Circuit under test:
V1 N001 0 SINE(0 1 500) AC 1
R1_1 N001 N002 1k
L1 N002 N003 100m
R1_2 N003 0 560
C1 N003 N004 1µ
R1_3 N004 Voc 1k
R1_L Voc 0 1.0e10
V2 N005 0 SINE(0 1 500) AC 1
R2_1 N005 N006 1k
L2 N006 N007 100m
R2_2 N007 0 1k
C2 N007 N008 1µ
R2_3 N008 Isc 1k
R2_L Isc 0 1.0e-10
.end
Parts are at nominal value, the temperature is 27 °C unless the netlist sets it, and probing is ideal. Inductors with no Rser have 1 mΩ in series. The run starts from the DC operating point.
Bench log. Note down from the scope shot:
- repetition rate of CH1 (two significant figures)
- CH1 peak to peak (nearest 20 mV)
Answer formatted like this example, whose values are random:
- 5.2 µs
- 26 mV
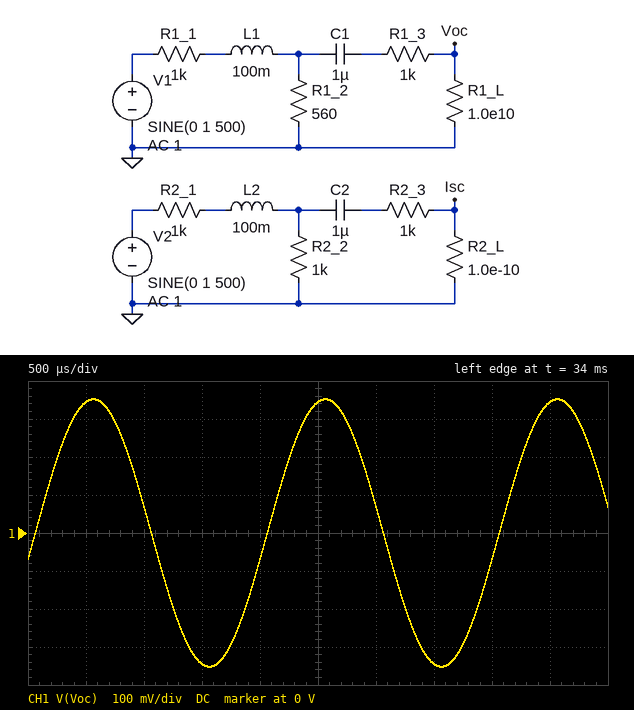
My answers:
- 500 Hz
- 700 mV
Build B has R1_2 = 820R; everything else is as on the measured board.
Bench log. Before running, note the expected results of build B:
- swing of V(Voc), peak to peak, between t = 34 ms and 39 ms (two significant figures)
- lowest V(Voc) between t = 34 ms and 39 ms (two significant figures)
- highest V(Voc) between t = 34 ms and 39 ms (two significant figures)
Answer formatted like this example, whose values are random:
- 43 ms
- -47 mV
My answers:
- 890 mV
- -440 mV
- 440 mV
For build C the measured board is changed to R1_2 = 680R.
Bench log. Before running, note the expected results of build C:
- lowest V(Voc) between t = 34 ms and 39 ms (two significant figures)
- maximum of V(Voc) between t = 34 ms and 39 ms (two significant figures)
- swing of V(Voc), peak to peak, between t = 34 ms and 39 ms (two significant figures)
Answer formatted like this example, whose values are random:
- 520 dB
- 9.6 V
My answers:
- -400 mV
- 400 mV
- 800 mV
